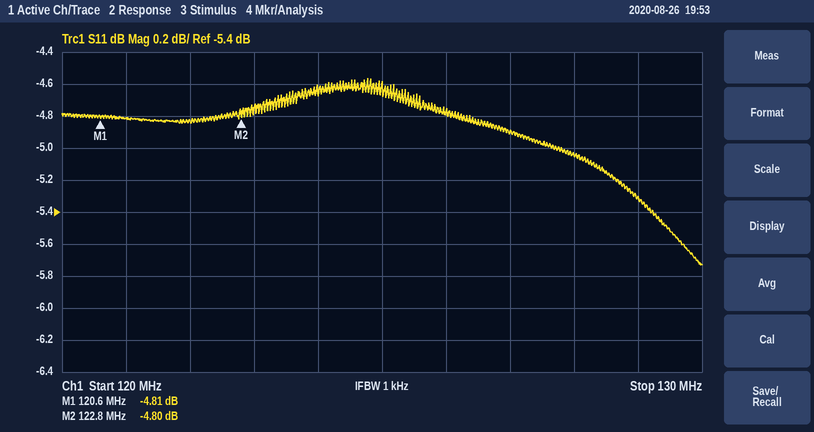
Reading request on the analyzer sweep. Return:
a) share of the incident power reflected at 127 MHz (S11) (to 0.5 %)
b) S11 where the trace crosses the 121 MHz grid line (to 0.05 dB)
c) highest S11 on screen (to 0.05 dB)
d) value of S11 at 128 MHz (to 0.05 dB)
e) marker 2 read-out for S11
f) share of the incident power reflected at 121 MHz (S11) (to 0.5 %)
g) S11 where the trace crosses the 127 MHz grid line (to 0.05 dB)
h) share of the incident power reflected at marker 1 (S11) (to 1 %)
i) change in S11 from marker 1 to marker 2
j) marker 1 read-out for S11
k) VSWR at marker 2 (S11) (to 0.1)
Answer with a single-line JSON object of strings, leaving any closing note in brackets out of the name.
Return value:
{"share of the incident power reflected at 127 MHz (S11)": "32.5 %", "S11 where the trace crosses the 121 MHz grid line": "-4.80 dB", "highest S11 on screen": "-4.55 dB", "value of S11 at 128 MHz": "-5.05 dB", "marker 2 read-out for S11": "-4.80 dB", "share of the incident power reflected at 121 MHz (S11)": "33.0 %", "S11 where the trace crosses the 127 MHz grid line": "-4.90 dB", "share of the incident power reflected at marker 1 (S11)": "33 %", "change in S11 from marker 1 to marker 2": "0.01 dB", "marker 1 read-out for S11": "-4.81 dB", "VSWR at marker 2 (S11)": "3.7"}
